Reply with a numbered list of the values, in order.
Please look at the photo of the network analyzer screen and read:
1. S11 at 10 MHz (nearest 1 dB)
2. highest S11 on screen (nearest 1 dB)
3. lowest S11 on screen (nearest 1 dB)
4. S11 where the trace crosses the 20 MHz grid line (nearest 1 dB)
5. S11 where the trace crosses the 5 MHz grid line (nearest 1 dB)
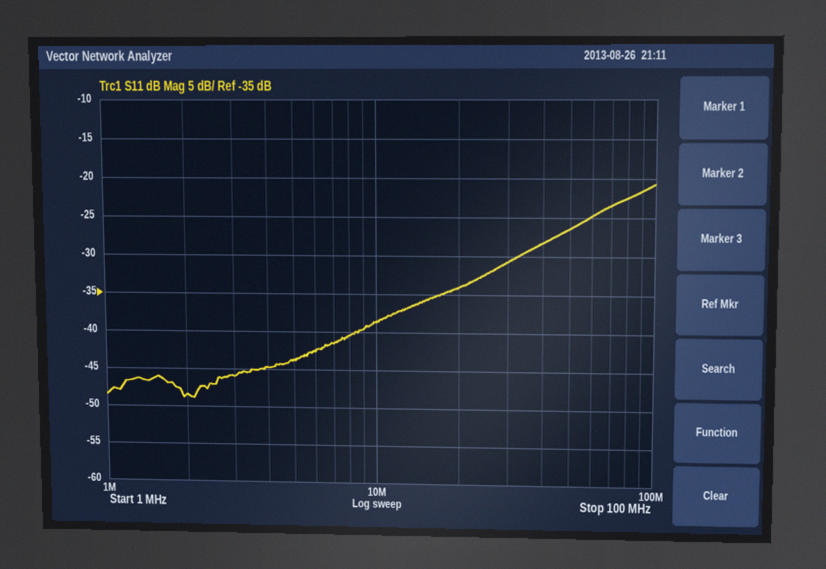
1. -39 dB
2. -21 dB
3. -49 dB
4. -34 dB
5. -44 dB
